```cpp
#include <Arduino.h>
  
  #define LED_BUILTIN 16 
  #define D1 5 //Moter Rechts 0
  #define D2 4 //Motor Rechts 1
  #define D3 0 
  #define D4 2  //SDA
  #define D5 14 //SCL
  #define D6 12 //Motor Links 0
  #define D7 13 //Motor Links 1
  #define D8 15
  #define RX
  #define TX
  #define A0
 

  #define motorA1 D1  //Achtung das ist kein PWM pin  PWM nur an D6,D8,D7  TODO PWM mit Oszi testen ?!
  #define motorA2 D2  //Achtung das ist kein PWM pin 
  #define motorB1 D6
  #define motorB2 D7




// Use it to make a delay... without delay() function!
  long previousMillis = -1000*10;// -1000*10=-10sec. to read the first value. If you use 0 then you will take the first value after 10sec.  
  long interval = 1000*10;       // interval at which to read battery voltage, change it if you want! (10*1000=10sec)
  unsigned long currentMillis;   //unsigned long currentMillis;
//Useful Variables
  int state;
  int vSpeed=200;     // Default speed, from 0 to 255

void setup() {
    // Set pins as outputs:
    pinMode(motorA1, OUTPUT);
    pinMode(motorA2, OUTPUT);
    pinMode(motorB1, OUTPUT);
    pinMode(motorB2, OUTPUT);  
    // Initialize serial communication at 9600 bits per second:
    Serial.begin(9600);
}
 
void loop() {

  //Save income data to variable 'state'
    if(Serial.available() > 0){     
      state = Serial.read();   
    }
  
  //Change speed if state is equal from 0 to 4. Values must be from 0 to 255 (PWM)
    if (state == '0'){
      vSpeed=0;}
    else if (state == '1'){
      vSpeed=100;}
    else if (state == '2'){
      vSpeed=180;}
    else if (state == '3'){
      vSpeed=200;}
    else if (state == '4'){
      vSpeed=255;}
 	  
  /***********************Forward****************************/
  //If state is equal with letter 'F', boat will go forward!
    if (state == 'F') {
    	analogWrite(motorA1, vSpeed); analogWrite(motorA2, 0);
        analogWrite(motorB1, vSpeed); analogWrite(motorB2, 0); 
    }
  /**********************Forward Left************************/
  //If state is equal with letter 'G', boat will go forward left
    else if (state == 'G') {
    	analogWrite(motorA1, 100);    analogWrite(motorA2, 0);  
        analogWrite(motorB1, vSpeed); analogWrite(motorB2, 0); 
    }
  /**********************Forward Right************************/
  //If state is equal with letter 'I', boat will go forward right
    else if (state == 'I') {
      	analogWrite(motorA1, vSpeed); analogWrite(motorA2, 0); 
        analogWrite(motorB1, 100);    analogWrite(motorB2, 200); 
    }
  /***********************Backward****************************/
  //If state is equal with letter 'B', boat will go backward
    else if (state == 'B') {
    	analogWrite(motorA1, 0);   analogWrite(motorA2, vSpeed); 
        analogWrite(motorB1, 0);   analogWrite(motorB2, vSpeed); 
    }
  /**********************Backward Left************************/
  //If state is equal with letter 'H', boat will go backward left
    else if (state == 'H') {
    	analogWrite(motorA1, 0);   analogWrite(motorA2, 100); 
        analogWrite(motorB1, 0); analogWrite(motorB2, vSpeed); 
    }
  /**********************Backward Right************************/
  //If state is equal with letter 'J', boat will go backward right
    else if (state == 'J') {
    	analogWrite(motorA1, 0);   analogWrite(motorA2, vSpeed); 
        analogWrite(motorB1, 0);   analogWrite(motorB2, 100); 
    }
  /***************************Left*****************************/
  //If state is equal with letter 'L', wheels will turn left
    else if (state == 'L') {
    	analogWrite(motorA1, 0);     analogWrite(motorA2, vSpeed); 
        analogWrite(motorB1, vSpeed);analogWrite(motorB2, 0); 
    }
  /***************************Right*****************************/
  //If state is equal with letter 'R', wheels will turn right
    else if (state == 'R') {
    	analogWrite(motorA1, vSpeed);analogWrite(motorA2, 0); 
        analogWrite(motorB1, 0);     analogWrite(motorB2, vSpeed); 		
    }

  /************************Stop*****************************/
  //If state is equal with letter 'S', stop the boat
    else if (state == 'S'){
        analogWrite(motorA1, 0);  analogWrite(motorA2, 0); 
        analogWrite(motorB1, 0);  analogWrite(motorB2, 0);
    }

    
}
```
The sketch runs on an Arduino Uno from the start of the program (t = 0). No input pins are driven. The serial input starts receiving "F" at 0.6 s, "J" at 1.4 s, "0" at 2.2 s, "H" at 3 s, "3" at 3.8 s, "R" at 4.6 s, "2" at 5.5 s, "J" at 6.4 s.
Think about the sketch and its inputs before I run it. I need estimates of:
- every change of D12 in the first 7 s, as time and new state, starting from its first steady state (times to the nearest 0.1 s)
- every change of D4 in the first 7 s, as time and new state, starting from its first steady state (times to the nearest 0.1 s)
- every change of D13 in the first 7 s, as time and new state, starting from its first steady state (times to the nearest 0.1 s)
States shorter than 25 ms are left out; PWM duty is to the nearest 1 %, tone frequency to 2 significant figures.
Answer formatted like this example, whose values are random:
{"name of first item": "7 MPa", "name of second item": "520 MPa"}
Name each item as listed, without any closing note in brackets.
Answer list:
{"every change of D12 in the first 7 s, as time and new state, starting from its first steady state": "0 s low; 0.6 s high; 1.4 s low", "every change of D4 in the first 7 s, as time and new state, starting from its first steady state": "0 s low; 1.4 s high; 3 s low; 6.4 s high", "every change of D13 in the first 7 s, as time and new state, starting from its first steady state": "0 s low; 4.6 s high; 6.4 s low"}
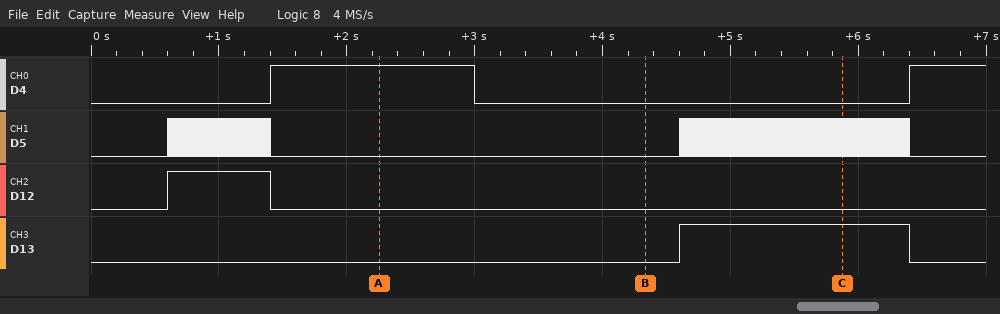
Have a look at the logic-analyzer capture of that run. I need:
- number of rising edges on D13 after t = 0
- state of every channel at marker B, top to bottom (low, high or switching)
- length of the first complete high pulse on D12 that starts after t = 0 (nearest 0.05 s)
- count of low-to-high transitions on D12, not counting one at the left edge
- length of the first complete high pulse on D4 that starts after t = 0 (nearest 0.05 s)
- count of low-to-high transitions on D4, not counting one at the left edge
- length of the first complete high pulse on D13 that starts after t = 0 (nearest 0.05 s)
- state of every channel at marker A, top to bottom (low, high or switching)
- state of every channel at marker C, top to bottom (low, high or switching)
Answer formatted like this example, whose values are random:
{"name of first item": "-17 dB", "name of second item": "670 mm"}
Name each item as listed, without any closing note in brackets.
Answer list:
{"number of rising edges on D13 after t = 0": "1", "state of every channel at marker B, top to bottom": "D4 low, D5 low, D12 low, D13 low", "length of the first complete high pulse on D12 that starts after t = 0": "0.80 s", "count of low-to-high transitions on D12, not counting one at the left edge": "1", "length of the first complete high pulse on D4 that starts after t = 0": "1.60 s", "count of low-to-high transitions on D4, not counting one at the left edge": "2", "length of the first complete high pulse on D13 that starts after t = 0": "1.80 s", "state of every channel at marker A, top to bottom": "D4 high, D5 low, D12 low, D13 low", "state of every channel at marker C, top to bottom": "D4 low, D5 switching, D12 low, D13 high"}
